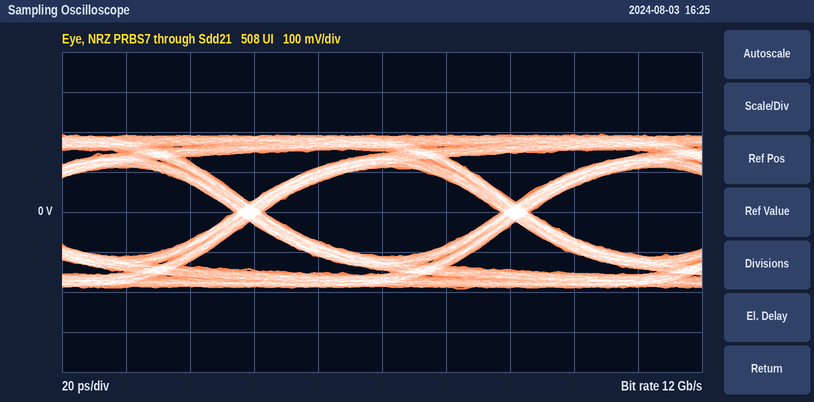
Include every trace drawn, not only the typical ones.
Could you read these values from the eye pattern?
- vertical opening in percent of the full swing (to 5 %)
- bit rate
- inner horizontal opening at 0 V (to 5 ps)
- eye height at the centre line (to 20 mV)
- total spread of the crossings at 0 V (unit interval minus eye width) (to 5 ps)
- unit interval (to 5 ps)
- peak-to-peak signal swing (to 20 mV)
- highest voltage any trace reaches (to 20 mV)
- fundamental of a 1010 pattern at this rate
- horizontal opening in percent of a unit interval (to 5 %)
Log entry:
60 %
12 Gb/s
75 ps
220 mV
10 ps
85 ps
380 mV
200 mV
6 GHz
90 %
